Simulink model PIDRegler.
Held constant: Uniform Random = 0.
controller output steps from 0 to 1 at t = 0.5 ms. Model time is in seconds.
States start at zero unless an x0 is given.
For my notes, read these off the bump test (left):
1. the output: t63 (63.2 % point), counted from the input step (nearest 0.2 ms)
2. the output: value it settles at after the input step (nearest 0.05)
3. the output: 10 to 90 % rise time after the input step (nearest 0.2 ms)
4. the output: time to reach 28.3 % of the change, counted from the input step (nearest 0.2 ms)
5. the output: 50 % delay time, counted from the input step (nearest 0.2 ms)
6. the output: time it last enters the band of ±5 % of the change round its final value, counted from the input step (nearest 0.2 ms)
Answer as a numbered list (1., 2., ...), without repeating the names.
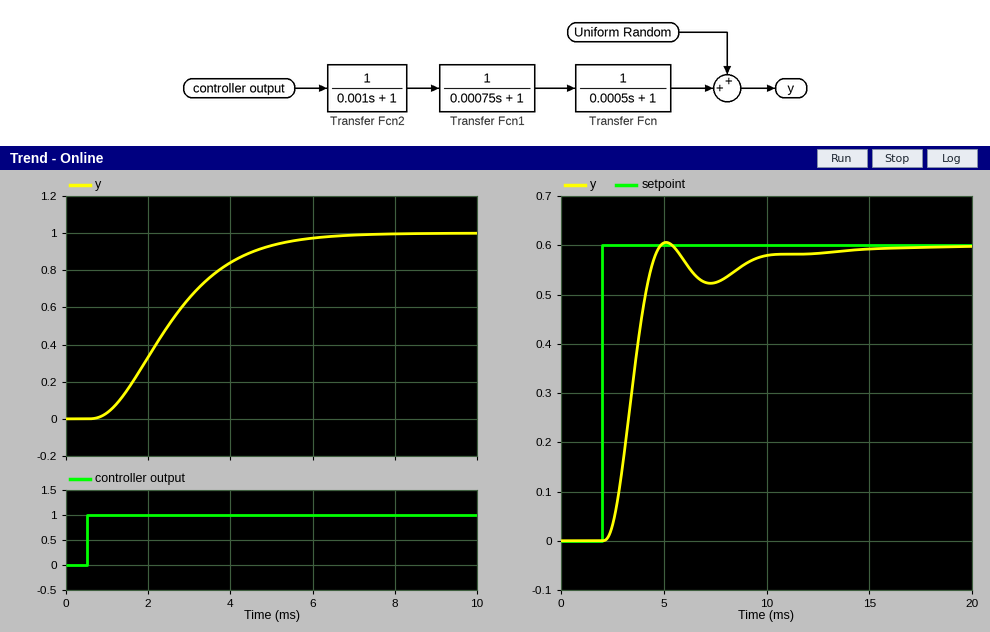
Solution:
1. 2.4 ms
2. 1.00
3. 3.2 ms
4. 1.4 ms
5. 2.0 ms
6. 4.8 ms
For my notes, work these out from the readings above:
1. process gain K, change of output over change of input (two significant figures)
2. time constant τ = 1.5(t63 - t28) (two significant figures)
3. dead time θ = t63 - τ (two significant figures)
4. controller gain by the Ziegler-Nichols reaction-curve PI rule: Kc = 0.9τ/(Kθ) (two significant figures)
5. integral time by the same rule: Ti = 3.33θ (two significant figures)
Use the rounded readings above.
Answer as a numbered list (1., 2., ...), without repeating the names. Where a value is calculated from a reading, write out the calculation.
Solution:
1. (1 - 0) / 1 = 1.0
2. 1.5 × (2.4 - 1.4) = 1.5 ms
3. 2.4 - 1.5 = 0.90 ms
4. 0.9 × 1.5 / (1 × 0.9) = 1.5
5. 3.33 × 0.9 = 3.0 ms
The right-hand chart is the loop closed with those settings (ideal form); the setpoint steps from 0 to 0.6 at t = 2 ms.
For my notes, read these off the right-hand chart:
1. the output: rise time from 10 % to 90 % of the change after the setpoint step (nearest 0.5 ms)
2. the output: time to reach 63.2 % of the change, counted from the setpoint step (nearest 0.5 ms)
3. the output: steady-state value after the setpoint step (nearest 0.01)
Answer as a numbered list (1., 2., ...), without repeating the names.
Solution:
1. 1.5 ms
2. 1.5 ms
3. 0.60
